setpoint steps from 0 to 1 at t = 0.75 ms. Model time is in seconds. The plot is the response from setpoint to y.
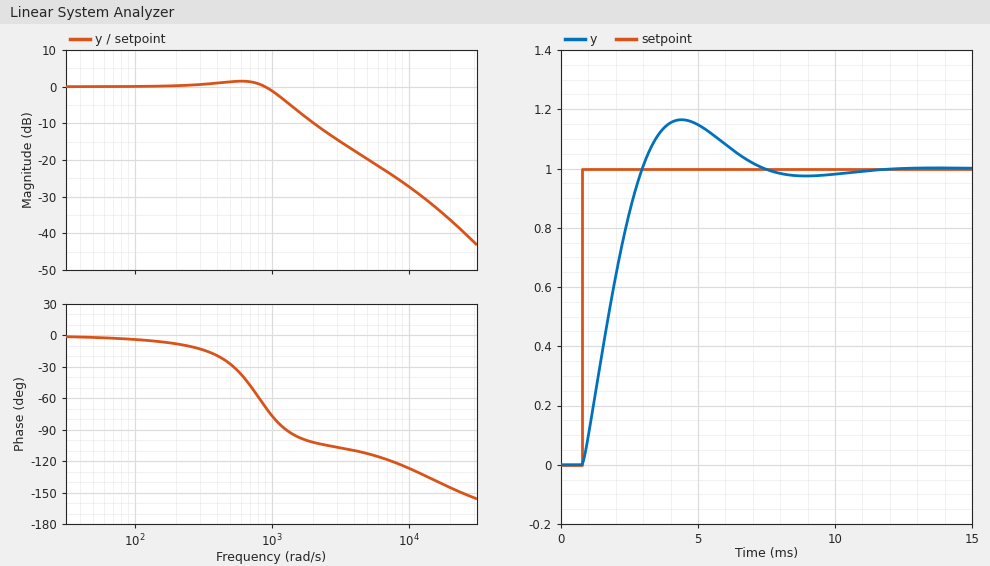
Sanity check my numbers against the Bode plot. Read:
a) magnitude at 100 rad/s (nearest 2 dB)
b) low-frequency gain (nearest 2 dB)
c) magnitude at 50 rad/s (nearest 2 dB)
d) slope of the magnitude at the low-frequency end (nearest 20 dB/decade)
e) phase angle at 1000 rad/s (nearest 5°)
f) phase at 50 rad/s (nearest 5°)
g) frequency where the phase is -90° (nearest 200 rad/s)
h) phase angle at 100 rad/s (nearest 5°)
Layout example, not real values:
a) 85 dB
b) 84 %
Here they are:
a) 0 dB
b) 0 dB
c) 0 dB
d) 0 dB/decade
e) -75°
f) 0°
g) 1200 rad/s
h) -5°
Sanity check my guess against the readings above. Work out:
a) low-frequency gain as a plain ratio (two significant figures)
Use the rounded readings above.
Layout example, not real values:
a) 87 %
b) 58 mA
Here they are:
a) 1.0
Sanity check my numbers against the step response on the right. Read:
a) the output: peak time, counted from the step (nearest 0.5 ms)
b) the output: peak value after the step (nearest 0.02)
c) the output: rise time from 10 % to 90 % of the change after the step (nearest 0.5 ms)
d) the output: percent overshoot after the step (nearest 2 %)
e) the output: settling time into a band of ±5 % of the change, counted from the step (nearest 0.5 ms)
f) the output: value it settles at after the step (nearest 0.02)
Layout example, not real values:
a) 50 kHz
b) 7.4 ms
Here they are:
a) 3.5 ms
b) 1.16
c) 1.5 ms
d) 16 %
e) 5.5 ms
f) 1.00
